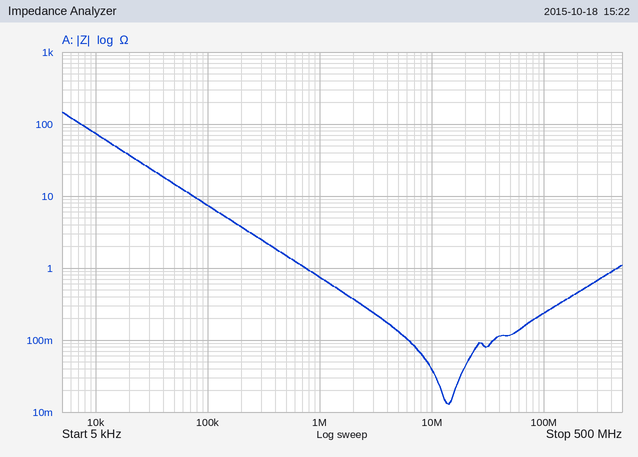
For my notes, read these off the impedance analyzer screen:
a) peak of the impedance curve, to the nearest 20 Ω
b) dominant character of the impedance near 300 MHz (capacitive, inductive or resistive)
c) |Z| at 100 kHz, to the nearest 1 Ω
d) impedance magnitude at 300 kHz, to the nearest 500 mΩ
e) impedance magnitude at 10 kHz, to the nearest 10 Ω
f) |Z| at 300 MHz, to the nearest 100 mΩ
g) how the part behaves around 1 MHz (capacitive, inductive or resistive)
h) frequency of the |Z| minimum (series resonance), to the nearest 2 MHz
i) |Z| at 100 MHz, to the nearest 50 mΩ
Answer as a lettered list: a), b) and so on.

a) 140 Ω
b) inductive
c) 7 Ω
d) 2.5 Ω
e) 70 Ω
f) 700 mΩ
g) capacitive
h) 14 MHz
i) 250 mΩ
